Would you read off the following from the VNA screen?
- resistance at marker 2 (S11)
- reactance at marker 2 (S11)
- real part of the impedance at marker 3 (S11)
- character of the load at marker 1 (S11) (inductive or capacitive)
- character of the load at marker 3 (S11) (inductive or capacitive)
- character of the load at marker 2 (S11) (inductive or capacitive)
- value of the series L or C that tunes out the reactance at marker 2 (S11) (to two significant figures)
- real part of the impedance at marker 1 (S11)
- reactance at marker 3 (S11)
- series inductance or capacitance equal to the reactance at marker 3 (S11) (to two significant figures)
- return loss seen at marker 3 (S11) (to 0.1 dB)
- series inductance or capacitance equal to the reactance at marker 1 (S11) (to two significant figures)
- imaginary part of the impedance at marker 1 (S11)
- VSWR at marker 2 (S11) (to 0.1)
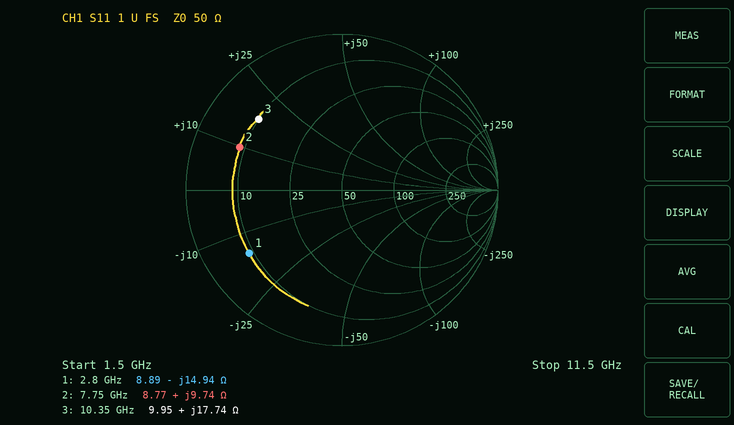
8.77 Ω
+9.74 Ω
9.95 Ω
capacitive
inductive
inductive
2.1 pF
8.89 Ω
+17.74 Ω
270 pH
3.1 dB
3.8 pF
-14.94 Ω
5.9
